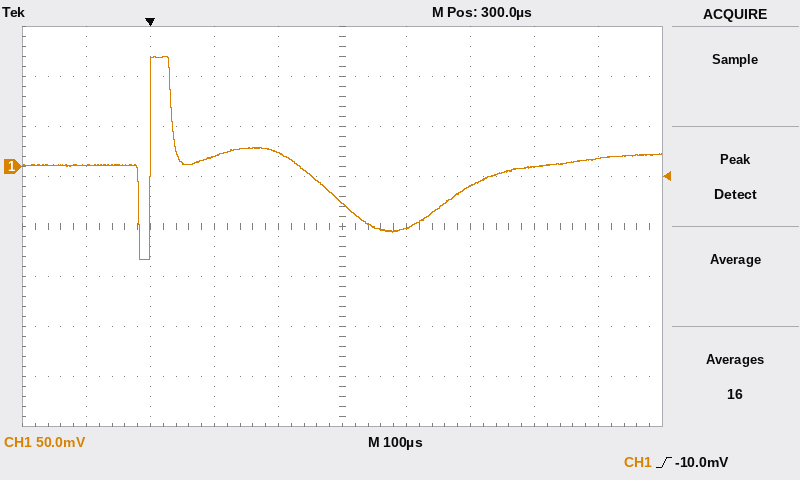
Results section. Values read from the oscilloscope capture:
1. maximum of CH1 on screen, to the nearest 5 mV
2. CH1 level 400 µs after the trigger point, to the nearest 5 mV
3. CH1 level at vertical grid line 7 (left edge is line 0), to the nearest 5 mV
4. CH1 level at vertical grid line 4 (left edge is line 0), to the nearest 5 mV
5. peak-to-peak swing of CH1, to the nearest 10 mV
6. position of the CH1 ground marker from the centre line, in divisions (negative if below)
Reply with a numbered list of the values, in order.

1. 110 mV
2. -60 mV
3. -20 mV
4. 15 mV
5. 200 mV
6. +1.2 div
